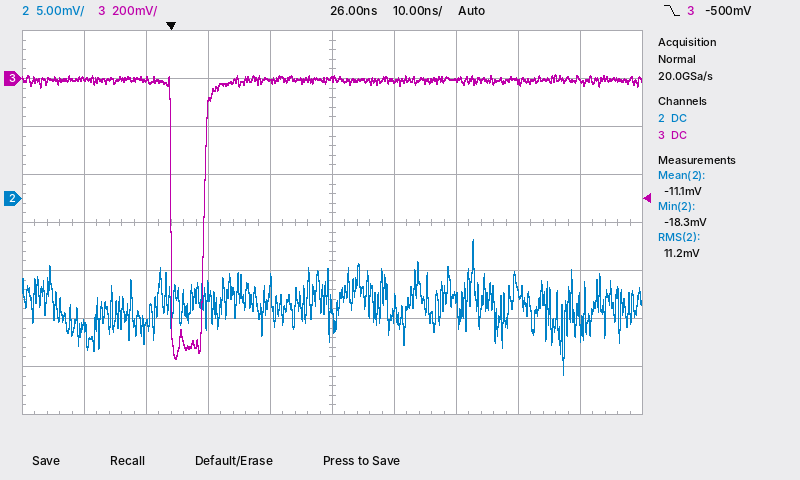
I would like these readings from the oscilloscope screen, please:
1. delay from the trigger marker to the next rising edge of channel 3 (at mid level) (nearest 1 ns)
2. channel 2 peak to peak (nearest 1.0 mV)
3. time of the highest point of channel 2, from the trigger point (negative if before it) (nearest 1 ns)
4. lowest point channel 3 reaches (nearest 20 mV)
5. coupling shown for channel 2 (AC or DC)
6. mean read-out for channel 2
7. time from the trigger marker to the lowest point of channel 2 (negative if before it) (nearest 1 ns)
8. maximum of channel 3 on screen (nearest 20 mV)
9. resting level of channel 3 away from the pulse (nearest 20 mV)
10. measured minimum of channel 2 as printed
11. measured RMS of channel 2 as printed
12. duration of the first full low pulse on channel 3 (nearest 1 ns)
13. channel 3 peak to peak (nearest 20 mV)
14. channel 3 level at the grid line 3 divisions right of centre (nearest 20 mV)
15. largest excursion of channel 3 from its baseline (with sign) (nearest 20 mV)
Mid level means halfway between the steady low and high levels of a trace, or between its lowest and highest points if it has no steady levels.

5 ns
14.0 mV
+49 ns
-1.16 V
DC
-11.1 mV
+63 ns
20 mV
0 mV
-18.3 mV
11.2 mV
5 ns
1.18 V
-20 mV
-1.16 V
